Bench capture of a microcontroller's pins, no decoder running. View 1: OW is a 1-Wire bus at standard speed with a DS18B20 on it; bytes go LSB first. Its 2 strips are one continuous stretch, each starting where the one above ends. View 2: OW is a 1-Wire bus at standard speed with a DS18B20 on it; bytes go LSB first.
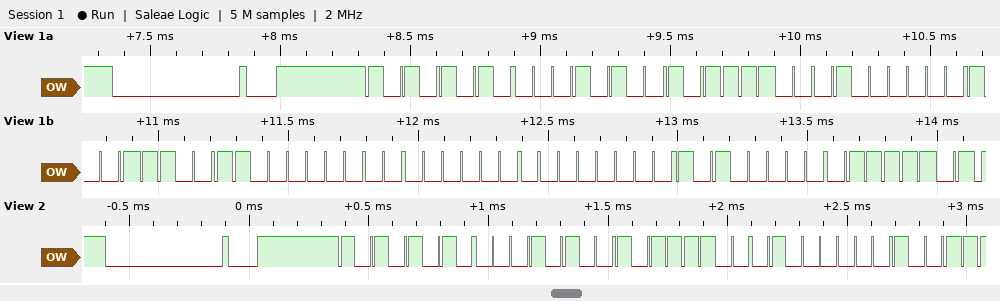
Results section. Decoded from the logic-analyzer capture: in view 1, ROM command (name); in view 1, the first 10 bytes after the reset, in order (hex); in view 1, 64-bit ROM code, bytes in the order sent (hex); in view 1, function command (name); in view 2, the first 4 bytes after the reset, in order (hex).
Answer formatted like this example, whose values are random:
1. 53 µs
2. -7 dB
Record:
1. Match ROM
2. 55 28 3D 02 39 03 00 00 05 BE
3. 28 3D 02 39 03 00 00 05
4. Read Scratchpad
5. 55 28 3D 02
